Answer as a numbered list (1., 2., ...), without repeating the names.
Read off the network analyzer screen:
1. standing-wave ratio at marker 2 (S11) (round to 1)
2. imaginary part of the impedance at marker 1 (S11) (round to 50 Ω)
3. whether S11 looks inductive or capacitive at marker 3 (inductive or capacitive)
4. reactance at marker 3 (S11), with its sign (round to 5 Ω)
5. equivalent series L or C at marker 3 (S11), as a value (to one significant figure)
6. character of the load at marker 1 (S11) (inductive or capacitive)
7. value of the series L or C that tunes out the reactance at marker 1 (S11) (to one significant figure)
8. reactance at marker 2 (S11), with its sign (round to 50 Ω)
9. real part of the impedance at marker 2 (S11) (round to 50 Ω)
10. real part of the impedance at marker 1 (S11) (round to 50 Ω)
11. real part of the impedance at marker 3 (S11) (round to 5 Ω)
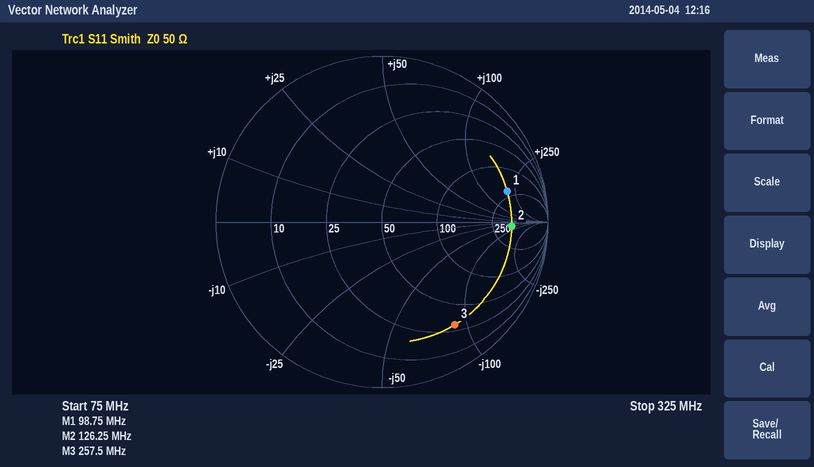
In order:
1. 8
2. +200 Ω
3. capacitive
4. -90 Ω
5. 7 pF
6. inductive
7. 8 pF
8. -50 Ω
9. 400 Ω
10. 200 Ω
11. 30 Ω
